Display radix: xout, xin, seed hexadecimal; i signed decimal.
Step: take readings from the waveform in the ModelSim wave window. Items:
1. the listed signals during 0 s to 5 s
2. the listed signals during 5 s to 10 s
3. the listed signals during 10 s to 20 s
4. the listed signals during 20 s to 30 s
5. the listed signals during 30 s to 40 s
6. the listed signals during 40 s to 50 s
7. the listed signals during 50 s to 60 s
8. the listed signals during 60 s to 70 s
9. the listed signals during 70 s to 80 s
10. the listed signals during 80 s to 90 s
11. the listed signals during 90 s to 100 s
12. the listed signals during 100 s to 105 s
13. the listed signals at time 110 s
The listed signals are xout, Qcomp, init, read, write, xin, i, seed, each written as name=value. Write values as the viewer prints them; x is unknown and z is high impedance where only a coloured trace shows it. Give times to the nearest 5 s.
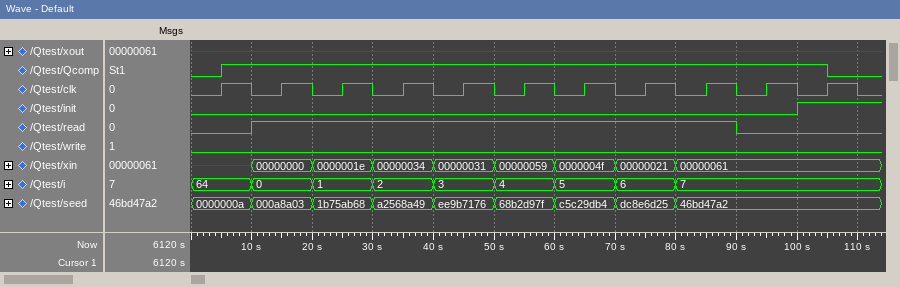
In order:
xout=x, Qcomp=0, init=0, read=0, write=0, xin=x, i=64, seed=0000000a
xout=x, Qcomp=1, init=0, read=0, write=0, xin=x, i=64, seed=0000000a
xout=x, Qcomp=1, init=0, read=1, write=0, xin=00000000, i=0, seed=000a8a03
xout=x, Qcomp=1, init=0, read=1, write=0, xin=0000001e, i=1, seed=1b75ab68
xout=x, Qcomp=1, init=0, read=1, write=0, xin=00000034, i=2, seed=a2568a49
xout=x, Qcomp=1, init=0, read=1, write=0, xin=00000031, i=3, seed=ee9b7176
xout=x, Qcomp=1, init=0, read=1, write=0, xin=00000059, i=4, seed=68b2d97f
xout=x, Qcomp=1, init=0, read=1, write=0, xin=0000004f, i=5, seed=c5c29db4
xout=x, Qcomp=1, init=0, read=1, write=0, xin=00000021, i=6, seed=dc8e6d25
xout=x, Qcomp=1, init=0, read=1, write=0, xin=00000061, i=7, seed=46bd47a2
xout=x, Qcomp=1, init=0, read=0, write=0, xin=00000061, i=7, seed=46bd47a2
xout=x, Qcomp=1, init=1, read=0, write=0, xin=00000061, i=7, seed=46bd47a2
xout=x, Qcomp=0, init=1, read=0, write=0, xin=00000061, i=7, seed=46bd47a2
